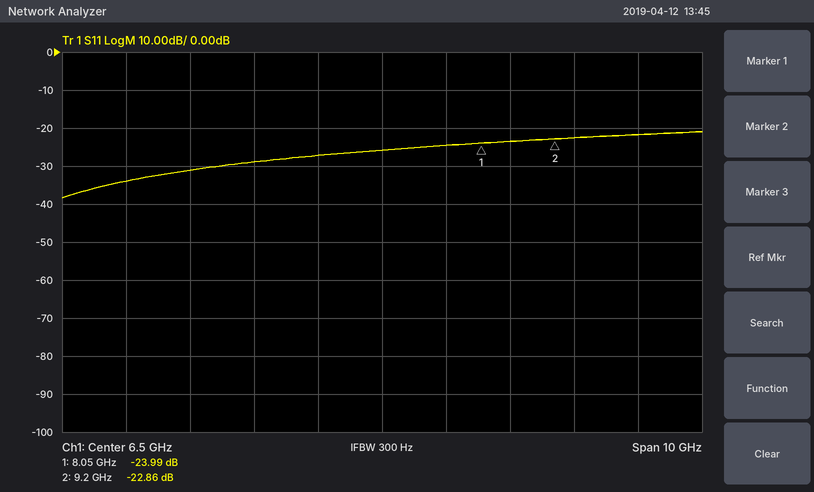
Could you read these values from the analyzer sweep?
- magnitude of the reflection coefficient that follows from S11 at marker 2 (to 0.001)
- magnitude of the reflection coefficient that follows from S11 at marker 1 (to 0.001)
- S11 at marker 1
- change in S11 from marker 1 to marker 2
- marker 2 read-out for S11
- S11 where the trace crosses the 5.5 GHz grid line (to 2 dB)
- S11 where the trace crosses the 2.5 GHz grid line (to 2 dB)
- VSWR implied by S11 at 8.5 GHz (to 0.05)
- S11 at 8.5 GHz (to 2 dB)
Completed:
0.072
0.063
-23.99 dB
1.13 dB
-22.86 dB
-28 dB
-34 dB
1.15
-24 dB
